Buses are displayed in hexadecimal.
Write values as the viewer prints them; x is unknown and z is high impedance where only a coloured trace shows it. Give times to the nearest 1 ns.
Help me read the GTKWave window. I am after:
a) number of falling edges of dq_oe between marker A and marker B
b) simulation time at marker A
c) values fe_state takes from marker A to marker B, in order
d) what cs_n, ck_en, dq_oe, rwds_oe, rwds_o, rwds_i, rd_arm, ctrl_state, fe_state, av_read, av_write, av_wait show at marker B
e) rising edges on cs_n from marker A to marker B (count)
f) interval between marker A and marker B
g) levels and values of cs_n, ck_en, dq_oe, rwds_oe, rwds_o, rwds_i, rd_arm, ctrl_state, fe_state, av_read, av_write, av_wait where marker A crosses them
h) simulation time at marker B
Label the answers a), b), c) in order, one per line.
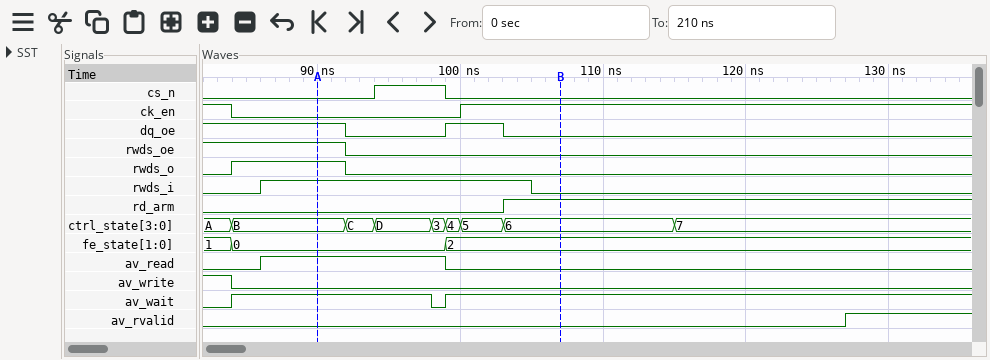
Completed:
a) 2
b) 90 ns
c) 0, 2
d) cs_n=0, ck_en=1, dq_oe=0, rwds_oe=0, rwds_o=0, rwds_i=0, rd_arm=1, ctrl_state=6, fe_state=2, av_read=0, av_write=0, av_wait=1
e) 1
f) 17 ns
g) cs_n=0, ck_en=0, dq_oe=1, rwds_oe=1, rwds_o=1, rwds_i=1, rd_arm=0, ctrl_state=B, fe_state=0, av_read=1, av_write=0, av_wait=1
h) 107 ns
